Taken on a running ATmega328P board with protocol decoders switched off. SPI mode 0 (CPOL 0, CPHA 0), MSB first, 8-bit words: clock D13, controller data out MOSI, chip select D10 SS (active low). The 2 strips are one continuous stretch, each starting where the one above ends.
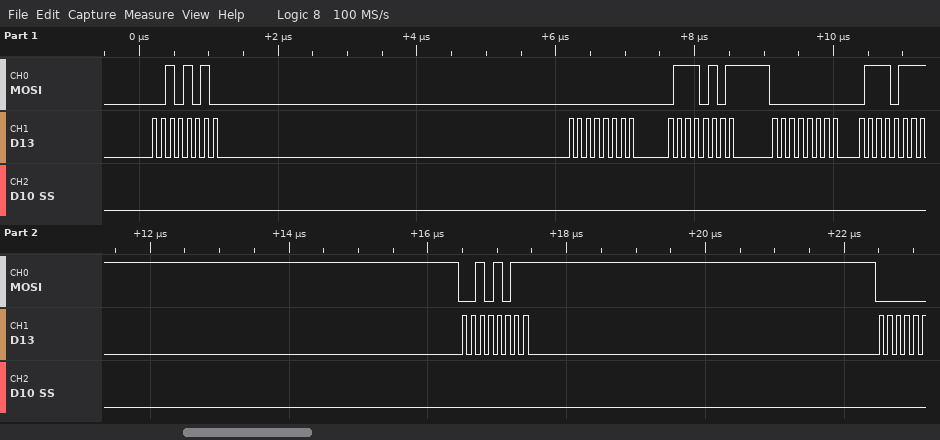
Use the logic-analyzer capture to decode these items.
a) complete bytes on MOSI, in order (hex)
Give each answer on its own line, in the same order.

0x2A 0x00 0x75 0x00 0x77 0x2B
